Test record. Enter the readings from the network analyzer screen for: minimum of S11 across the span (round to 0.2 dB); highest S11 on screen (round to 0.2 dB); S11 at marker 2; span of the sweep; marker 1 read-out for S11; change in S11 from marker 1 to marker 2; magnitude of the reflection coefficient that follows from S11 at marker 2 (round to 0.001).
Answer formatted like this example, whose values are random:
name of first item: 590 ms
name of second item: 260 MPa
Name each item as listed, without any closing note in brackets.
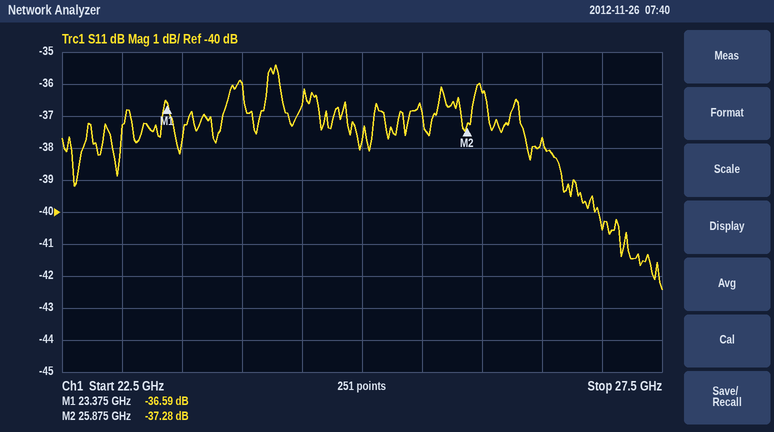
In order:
minimum of S11 across the span: -42.4 dB
highest S11 on screen: -35.4 dB
S11 at marker 2: -37.28 dB
span of the sweep: 5 GHz
marker 1 read-out for S11: -36.59 dB
change in S11 from marker 1 to marker 2: -0.69 dB
magnitude of the reflection coefficient that follows from S11 at marker 2: 0.014
